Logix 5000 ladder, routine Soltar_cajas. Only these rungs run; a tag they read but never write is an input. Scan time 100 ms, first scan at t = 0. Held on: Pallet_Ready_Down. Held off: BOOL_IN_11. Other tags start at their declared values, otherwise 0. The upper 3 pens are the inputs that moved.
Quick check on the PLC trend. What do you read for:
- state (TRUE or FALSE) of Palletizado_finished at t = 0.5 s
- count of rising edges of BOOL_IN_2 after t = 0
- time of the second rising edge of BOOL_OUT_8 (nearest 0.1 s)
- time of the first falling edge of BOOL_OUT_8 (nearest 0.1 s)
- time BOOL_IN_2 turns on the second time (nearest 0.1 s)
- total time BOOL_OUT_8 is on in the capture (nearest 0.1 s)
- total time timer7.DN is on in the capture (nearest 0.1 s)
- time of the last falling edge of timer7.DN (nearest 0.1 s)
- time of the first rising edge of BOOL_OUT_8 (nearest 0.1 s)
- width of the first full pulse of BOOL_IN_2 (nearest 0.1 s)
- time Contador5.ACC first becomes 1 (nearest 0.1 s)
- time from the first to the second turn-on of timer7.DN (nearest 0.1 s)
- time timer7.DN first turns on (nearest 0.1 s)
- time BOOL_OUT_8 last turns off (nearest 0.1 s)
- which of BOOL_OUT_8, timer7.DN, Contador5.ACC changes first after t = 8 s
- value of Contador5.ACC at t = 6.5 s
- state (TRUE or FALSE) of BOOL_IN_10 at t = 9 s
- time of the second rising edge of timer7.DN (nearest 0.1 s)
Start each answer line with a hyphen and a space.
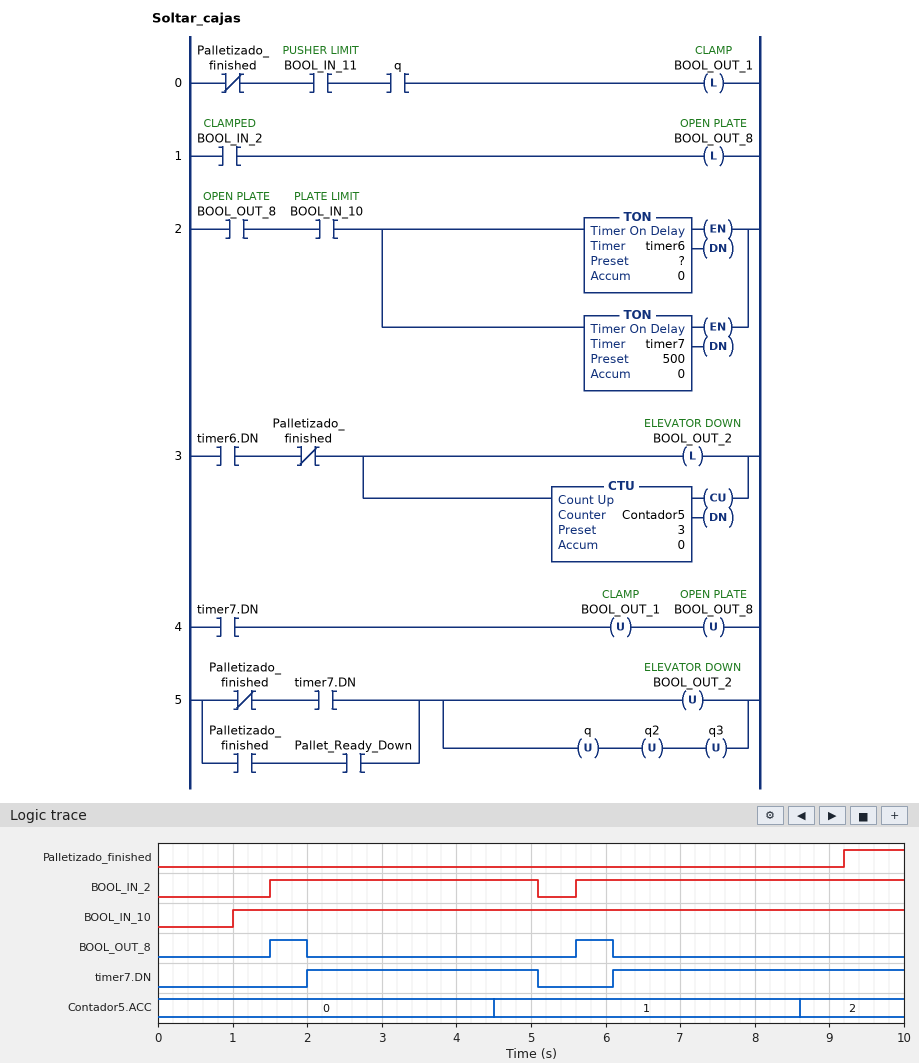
- FALSE
- 2
- 5.6 s
- 2.0 s
- 5.6 s
- 1.0 s
- 7.0 s
- 5.1 s
- 1.5 s
- 3.6 s
- 4.5 s
- 4.1 s
- 2.0 s
- 6.1 s
- Contador5.ACC
- 1
- TRUE
- 6.1 s
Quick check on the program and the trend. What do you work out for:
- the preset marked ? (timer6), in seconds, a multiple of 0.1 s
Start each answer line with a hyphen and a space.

- 3.0 s
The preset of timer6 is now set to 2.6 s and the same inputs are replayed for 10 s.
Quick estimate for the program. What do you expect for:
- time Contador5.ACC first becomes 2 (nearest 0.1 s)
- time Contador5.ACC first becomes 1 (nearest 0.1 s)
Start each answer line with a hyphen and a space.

- 8.2 s
- 4.1 s
